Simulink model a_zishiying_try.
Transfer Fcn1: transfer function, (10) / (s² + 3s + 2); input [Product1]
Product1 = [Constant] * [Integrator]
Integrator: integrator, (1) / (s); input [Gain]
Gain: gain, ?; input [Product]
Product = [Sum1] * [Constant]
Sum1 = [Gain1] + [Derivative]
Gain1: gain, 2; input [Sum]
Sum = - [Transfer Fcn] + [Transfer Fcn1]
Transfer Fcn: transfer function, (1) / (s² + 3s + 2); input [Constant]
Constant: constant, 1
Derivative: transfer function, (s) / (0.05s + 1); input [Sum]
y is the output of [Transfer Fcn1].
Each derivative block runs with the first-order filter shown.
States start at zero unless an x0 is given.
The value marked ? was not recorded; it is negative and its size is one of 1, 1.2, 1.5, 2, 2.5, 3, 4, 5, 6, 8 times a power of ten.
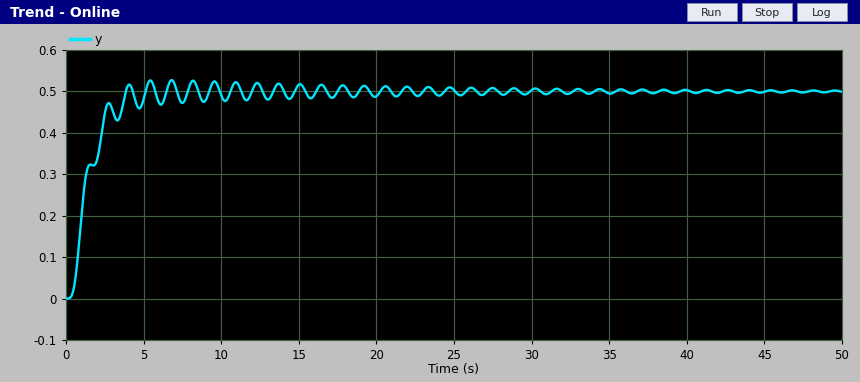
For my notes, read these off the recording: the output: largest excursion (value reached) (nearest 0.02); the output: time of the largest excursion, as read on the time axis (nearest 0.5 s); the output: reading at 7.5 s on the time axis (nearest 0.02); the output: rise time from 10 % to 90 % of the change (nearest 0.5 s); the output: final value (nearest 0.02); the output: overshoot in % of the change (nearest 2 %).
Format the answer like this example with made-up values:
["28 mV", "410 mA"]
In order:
["0.52", "7.0 s", "0.48", "2.0 s", "0.50", "6 %"]
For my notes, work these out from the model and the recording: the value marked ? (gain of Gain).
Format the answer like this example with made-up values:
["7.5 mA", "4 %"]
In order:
["-2"]
